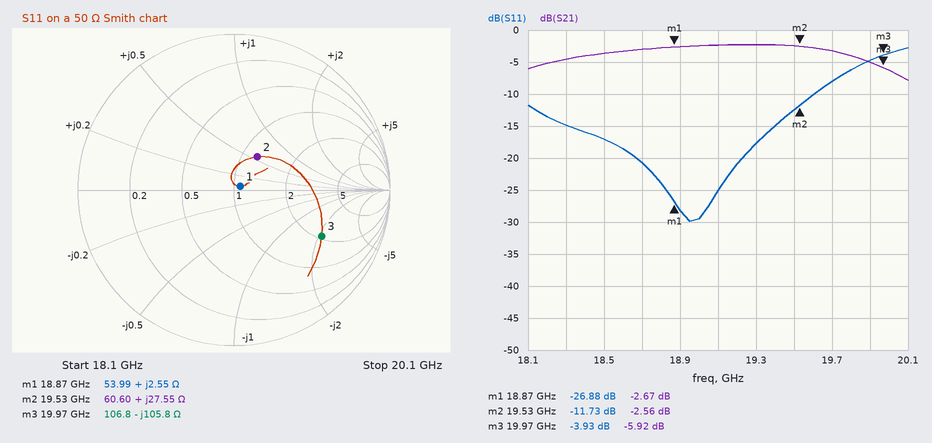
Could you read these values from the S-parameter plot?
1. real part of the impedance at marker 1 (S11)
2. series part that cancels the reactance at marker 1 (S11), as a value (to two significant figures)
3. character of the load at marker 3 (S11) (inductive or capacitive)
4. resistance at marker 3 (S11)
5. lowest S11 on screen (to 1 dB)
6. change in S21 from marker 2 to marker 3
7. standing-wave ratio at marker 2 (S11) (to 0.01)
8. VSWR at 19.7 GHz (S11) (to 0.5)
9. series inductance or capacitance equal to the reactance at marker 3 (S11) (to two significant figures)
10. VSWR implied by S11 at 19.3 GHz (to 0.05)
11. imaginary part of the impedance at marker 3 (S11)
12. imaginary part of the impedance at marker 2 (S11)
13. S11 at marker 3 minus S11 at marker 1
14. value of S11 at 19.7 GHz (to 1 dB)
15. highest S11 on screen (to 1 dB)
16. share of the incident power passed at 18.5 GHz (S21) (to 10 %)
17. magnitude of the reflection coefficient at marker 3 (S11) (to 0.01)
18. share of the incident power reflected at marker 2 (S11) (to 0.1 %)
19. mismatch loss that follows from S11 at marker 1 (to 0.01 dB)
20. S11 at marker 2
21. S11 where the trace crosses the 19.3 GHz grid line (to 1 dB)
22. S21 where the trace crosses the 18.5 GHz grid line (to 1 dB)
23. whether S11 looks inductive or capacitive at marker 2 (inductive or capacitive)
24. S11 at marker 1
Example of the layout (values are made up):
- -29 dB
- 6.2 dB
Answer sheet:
- 53.99 Ω
- 3.3 pF
- capacitive
- 106.8 Ω
- -30 dB
- -3.36 dB
- 1.70
- 2.5
- 75 fF
- 1.30
- -105.8 Ω
- +27.55 Ω
- 22.95 dB
- -8 dB
- -3 dB
- 40 %
- 0.64
- 6.7 %
- 0.01 dB
- -11.73 dB
- -18 dB
- -4 dB
- inductive
- -26.88 dB
